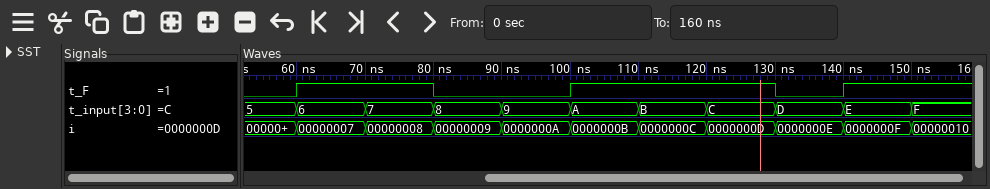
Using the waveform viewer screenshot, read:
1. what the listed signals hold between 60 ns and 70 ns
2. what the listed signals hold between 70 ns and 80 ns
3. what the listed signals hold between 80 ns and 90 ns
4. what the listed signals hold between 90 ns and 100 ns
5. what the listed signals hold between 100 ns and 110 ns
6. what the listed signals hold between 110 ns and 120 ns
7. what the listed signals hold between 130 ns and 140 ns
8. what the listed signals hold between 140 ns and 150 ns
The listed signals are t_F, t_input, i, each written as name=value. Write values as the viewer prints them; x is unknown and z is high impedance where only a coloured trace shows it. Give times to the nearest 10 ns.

t_F=1, t_input=6, i=00000007
t_F=1, t_input=7, i=00000008
t_F=0, t_input=8, i=00000009
t_F=0, t_input=9, i=0000000A
t_F=1, t_input=A, i=0000000B
t_F=1, t_input=B, i=0000000C
t_F=0, t_input=D, i=0000000E
t_F=1, t_input=E, i=0000000F
